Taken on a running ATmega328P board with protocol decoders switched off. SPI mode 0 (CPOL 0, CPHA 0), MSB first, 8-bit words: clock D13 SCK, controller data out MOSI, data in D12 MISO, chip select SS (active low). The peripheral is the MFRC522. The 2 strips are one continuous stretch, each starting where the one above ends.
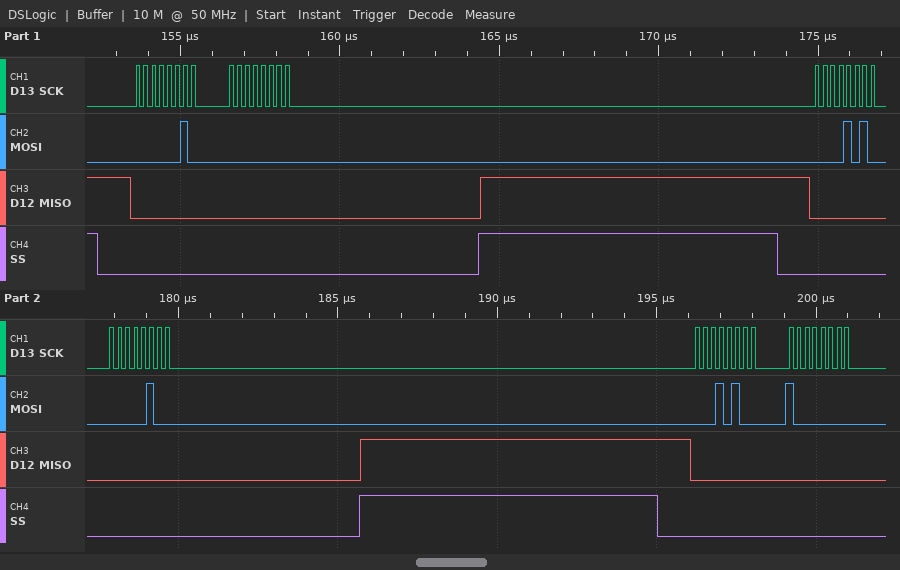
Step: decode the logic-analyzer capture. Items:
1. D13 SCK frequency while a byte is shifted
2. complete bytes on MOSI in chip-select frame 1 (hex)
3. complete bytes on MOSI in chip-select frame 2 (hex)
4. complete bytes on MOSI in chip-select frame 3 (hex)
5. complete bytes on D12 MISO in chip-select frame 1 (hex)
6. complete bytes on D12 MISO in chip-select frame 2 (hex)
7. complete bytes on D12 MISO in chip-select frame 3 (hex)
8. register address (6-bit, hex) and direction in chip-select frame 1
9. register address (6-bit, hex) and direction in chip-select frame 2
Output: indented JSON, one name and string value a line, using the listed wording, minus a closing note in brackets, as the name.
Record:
{
  "D13 SCK frequency while a byte is shifted": "4 MHz",
  "complete bytes on MOSI in chip-select frame 1": "02 00",
  "complete bytes on MOSI in chip-select frame 2": "0A 04",
  "complete bytes on MOSI in chip-select frame 3": "14 80",
  "complete bytes on D12 MISO in chip-select frame 1": "00 00",
  "complete bytes on D12 MISO in chip-select frame 2": "00 00",
  "complete bytes on D12 MISO in chip-select frame 3": "00 00",
  "register address (6-bit, hex) and direction in chip-select frame 1": "0x01 write",
  "register address (6-bit, hex) and direction in chip-select frame 2": "0x05 write"
}
